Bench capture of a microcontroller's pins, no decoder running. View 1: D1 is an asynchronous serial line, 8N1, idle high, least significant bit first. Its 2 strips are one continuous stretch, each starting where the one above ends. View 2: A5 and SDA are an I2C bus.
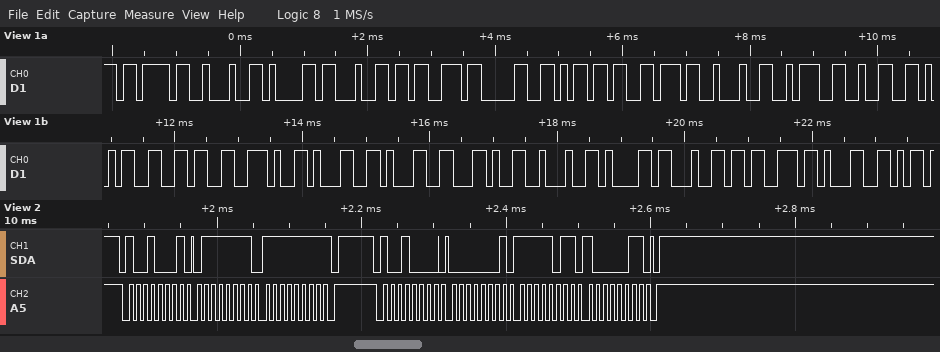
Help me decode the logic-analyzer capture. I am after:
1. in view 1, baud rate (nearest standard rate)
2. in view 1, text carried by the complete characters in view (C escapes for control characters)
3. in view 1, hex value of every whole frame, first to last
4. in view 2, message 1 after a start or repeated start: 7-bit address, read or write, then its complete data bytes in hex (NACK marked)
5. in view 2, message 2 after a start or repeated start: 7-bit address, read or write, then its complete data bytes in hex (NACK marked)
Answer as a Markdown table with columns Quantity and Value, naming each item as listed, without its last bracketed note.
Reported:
| Quantity | Value |
|---|---|
| in view 1, baud rate | 9600 baud |
| in view 1, text carried by the complete characters in view | "{\"ads0mv\":256.11,\"ads1" |
| in view 1, hex value of every whole frame, first to last | 7B 22 61 64 73 30 6D 76 22 3A 32 35 36 2E 31 31 2C 22 61 64 73 31 |
| in view 2, message 1 after a start or repeated start: 7-bit address, read or write, then its complete data bytes in hex | 0x48 read: 7F FF NACK |
| in view 2, message 2 after a start or repeated start: 7-bit address, read or write, then its complete data bytes in hex | 0x48 write: 01 FB 83 |
